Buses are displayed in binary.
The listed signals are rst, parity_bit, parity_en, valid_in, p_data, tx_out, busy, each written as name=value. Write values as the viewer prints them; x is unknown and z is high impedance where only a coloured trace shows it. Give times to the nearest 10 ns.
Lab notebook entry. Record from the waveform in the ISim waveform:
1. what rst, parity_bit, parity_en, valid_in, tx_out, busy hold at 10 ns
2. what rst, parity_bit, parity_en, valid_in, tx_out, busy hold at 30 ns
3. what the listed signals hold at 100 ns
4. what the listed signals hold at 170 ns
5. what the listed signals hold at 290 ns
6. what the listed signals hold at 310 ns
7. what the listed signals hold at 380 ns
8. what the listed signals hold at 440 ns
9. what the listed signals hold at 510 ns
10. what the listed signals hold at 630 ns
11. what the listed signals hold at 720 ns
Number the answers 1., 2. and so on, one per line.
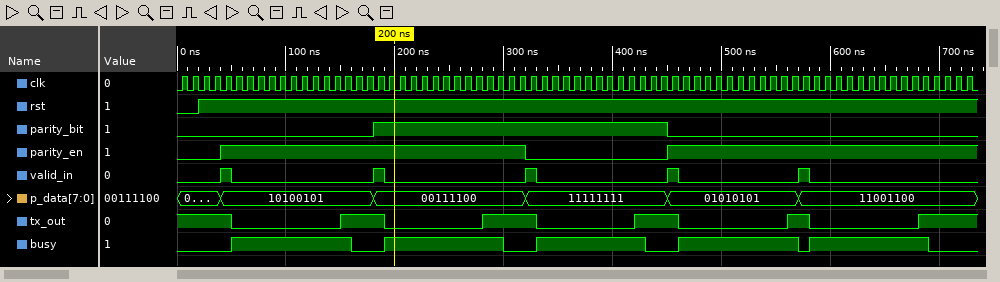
1. rst=0, parity_bit=0, parity_en=0, valid_in=0, tx_out=1, busy=0
2. rst=1, parity_bit=0, parity_en=0, valid_in=0, tx_out=1, busy=0
3. rst=1, parity_bit=0, parity_en=1, valid_in=0, p_data=10100101, tx_out=0, busy=1
4. rst=1, parity_bit=0, parity_en=1, valid_in=0, p_data=10100101, tx_out=1, busy=0
5. rst=1, parity_bit=1, parity_en=1, valid_in=0, p_data=00111100, tx_out=1, busy=1
6. rst=1, parity_bit=1, parity_en=1, valid_in=0, p_data=00111100, tx_out=1, busy=0
7. rst=1, parity_bit=1, parity_en=0, valid_in=0, p_data=11111111, tx_out=0, busy=1
8. rst=1, parity_bit=1, parity_en=0, valid_in=0, p_data=11111111, tx_out=1, busy=0
9. rst=1, parity_bit=0, parity_en=1, valid_in=0, p_data=01010101, tx_out=0, busy=1
10. rst=1, parity_bit=0, parity_en=1, valid_in=0, p_data=11001100, tx_out=0, busy=1
11. rst=1, parity_bit=0, parity_en=1, valid_in=0, p_data=11001100, tx_out=1, busy=0
